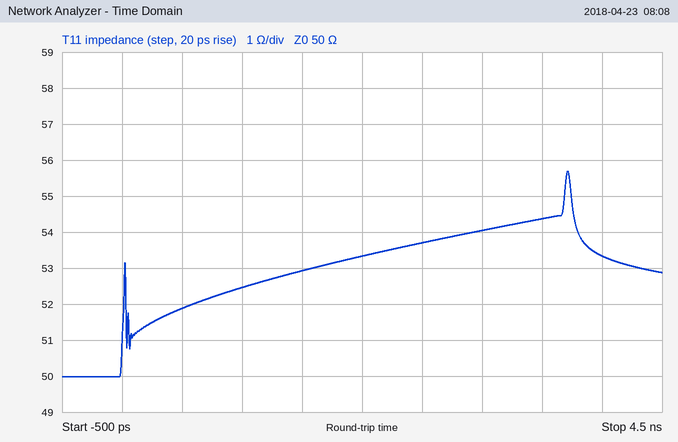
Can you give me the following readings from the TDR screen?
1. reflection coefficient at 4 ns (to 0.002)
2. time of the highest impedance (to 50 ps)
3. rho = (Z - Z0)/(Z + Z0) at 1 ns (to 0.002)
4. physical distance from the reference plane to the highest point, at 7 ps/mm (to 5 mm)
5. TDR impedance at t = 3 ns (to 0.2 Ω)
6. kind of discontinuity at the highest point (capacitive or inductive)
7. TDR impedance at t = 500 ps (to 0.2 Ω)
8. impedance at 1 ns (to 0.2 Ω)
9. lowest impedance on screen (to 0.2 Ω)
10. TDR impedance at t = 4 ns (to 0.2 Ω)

+0.032
3.70 ns
+0.024
265 mm
54.0 Ω
inductive
51.8 Ω
52.4 Ω
50.0 Ω
53.4 Ω
